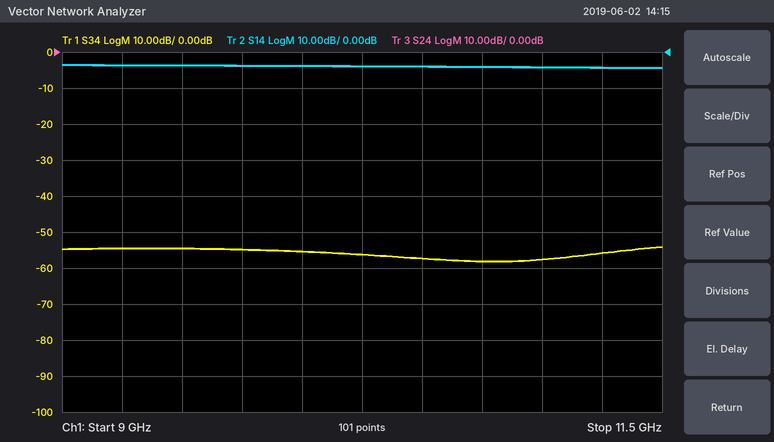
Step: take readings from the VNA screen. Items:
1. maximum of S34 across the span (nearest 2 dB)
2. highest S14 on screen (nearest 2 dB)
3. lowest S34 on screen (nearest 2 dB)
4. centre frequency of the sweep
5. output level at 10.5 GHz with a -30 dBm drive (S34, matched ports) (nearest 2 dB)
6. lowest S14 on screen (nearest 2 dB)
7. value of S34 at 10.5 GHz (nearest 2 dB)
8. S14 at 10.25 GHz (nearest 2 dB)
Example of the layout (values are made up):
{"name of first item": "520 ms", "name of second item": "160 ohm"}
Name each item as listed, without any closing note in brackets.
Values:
{"maximum of S34 across the span": "-54 dB", "highest S14 on screen": "-4 dB", "lowest S34 on screen": "-58 dB", "centre frequency of the sweep": "10.25 GHz", "output level at 10.5 GHz with a -30 dBm drive (S34, matched ports)": "-88 dBm", "lowest S14 on screen": "-4 dB", "value of S34 at 10.5 GHz": "-58 dB", "S14 at 10.25 GHz": "-4 dB"}
